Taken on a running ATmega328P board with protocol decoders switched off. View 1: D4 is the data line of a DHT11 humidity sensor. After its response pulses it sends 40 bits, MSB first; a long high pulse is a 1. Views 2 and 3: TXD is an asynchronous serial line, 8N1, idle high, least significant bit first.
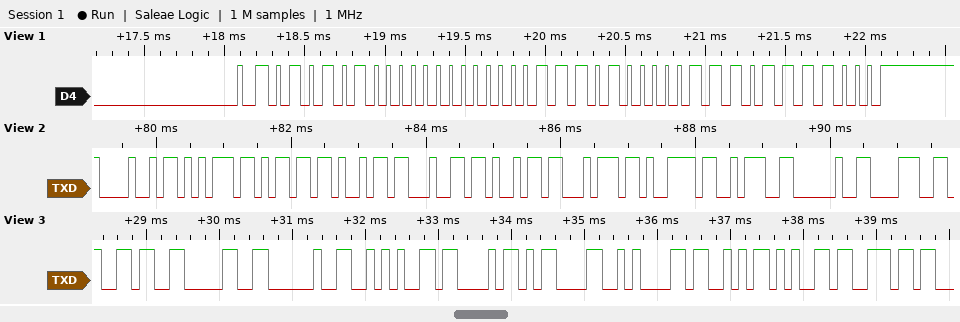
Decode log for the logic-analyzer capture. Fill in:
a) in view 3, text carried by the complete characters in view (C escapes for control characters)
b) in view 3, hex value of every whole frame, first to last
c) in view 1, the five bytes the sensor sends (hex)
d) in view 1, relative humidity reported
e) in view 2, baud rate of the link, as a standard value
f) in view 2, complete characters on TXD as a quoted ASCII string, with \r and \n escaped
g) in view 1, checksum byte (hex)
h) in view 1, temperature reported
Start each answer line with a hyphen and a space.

- "60 *C\r\nSen"
- 36 30 20 2A 43 0D 0A 53 65 6E
- 54 00 1D 07 78
- 84 %
- 9600 baud
- "Humidity: 8"
- 0x78
- 29.7 °C
